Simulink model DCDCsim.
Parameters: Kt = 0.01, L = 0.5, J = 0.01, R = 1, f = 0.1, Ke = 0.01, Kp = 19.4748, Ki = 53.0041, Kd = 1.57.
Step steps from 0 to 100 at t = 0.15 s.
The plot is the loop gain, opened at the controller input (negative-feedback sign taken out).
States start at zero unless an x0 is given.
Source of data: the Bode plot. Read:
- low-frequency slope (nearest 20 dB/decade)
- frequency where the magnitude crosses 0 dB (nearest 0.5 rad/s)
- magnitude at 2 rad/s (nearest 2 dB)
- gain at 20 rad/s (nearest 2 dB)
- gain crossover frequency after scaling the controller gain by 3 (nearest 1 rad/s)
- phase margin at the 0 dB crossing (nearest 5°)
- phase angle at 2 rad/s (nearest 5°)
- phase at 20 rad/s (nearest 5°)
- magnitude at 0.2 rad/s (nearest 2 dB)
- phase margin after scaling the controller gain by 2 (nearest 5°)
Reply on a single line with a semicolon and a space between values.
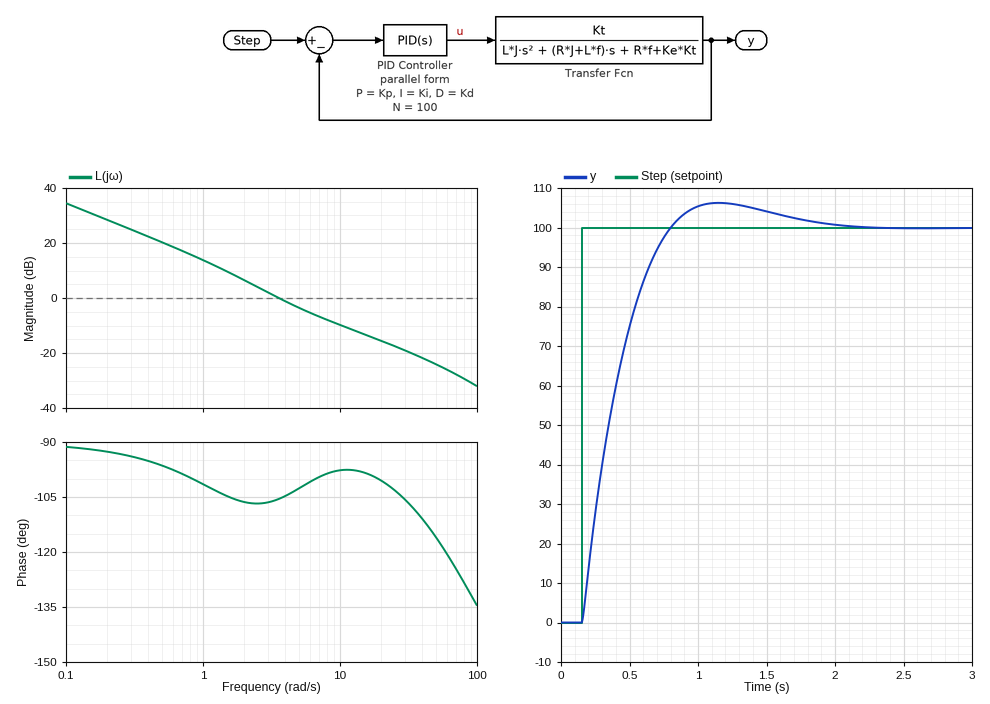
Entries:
-20 dB/decade; 3.5 rad/s; 6 dB; -16 dB; 10 rad/s; 75°; -105°; -100°; 28 dB; 80°
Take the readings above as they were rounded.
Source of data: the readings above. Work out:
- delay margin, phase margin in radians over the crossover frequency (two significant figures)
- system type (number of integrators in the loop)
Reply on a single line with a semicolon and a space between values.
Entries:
0.37 s; 1
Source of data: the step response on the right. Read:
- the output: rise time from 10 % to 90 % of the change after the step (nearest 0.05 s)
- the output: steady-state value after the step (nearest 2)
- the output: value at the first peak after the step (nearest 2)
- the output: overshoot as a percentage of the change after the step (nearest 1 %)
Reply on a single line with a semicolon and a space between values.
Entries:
0.45 s; 100; 106; 6 %
